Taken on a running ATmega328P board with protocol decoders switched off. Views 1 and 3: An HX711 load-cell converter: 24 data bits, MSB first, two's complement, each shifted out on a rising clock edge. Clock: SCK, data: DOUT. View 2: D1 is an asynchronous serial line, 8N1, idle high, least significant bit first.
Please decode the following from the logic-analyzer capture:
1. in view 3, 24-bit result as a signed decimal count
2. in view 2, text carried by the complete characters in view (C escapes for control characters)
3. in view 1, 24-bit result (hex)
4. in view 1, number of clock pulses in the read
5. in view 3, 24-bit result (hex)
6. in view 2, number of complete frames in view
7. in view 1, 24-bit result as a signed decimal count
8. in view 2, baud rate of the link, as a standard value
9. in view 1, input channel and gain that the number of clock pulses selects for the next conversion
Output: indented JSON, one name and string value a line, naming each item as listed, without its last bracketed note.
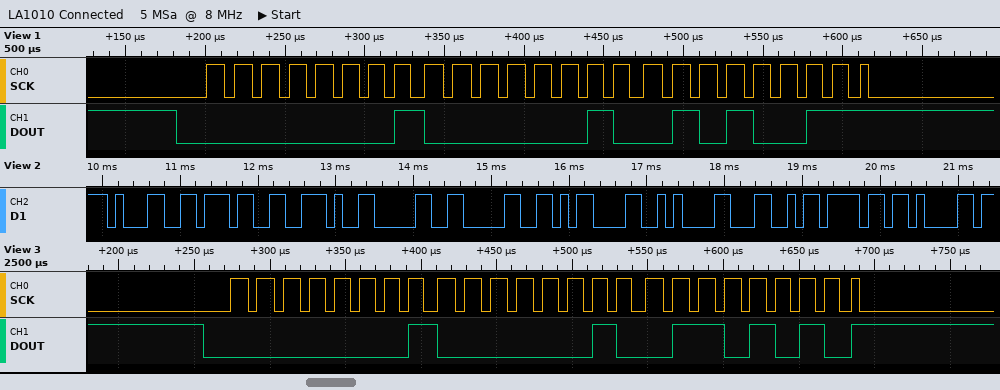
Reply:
{
  "in view 3, 24-bit result as a signed decimal count": "66154",
  "in view 2, text carried by the complete characters in view": "\"17.00\\r\\nLoa\"",
  "in view 1, 24-bit result": "0x010253",
  "in view 1, number of clock pulses in the read": "25",
  "in view 3, 24-bit result": "0x01026A",
  "in view 2, number of complete frames in view": "10",
  "in view 1, 24-bit result as a signed decimal count": "66131",
  "in view 2, baud rate of the link, as a standard value": "9600 baud",
  "in view 1, input channel and gain that the number of clock pulses selects for the next conversion": "channel A, gain 128"
}
